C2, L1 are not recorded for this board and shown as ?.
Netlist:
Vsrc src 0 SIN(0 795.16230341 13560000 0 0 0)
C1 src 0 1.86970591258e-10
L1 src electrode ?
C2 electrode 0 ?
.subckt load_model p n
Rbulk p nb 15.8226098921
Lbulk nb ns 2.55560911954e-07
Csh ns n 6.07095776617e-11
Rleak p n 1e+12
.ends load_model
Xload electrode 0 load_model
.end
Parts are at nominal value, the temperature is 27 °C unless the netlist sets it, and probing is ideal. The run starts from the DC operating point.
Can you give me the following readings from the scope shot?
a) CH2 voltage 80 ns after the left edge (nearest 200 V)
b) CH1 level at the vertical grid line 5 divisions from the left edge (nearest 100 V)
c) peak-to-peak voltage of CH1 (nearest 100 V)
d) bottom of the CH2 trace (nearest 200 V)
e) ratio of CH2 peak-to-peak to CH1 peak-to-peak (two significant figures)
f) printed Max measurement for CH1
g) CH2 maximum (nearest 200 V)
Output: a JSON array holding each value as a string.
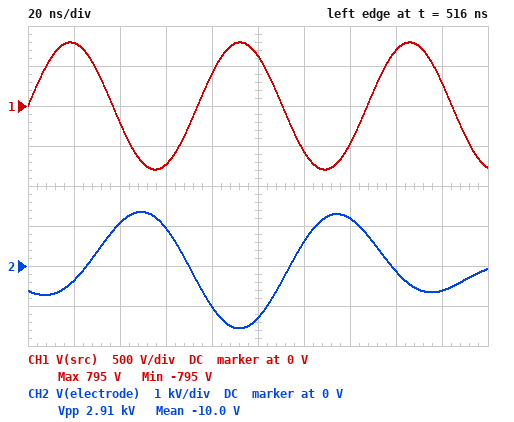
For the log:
["-1.0 kV", "600 V", "1.6 kV", "-1.6 kV", "1.8", "795 V", "1.4 kV"]
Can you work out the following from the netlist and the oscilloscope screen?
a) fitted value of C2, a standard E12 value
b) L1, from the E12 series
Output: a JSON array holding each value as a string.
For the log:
["220 pF", "1 µH"]
